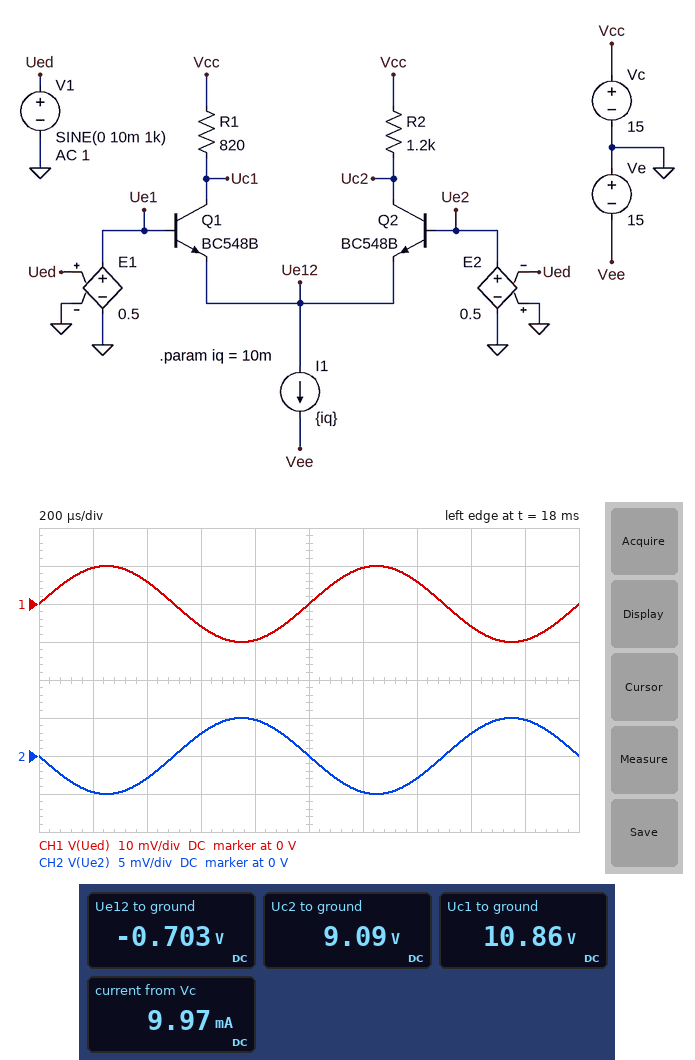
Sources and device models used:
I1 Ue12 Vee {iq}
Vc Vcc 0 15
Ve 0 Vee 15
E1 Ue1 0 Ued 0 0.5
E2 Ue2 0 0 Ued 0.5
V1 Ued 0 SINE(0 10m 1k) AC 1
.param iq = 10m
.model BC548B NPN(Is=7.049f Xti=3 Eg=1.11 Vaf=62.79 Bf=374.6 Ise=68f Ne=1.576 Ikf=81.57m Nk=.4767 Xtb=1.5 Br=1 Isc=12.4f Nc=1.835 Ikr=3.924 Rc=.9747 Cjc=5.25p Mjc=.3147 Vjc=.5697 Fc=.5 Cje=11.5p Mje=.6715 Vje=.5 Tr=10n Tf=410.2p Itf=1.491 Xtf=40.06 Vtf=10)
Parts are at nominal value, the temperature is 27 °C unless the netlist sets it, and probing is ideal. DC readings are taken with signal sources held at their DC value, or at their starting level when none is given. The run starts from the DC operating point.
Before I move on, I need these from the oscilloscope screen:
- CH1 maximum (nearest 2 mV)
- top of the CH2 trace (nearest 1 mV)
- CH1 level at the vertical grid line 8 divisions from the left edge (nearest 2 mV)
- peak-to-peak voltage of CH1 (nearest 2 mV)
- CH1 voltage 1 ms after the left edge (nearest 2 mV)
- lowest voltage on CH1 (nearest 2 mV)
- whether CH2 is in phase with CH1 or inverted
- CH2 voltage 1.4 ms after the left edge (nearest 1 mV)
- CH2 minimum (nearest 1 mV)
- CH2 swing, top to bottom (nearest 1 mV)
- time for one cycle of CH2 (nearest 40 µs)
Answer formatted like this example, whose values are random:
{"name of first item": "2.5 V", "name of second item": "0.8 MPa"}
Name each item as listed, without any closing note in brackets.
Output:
{"CH1 maximum": "10 mV", "top of the CH2 trace": "5 mV", "CH1 level at the vertical grid line 8 divisions from the left edge": "-6 mV", "peak-to-peak voltage of CH1": "20 mV", "CH1 voltage 1 ms after the left edge": "0 V", "lowest voltage on CH1": "-10 mV", "whether CH2 is in phase with CH1 or inverted": "inverted", "CH2 voltage 1.4 ms after the left edge": "-3 mV", "CH2 minimum": "-5 mV", "CH2 swing, top to bottom": "10 mV", "time for one cycle of CH2": "1.00 ms"}
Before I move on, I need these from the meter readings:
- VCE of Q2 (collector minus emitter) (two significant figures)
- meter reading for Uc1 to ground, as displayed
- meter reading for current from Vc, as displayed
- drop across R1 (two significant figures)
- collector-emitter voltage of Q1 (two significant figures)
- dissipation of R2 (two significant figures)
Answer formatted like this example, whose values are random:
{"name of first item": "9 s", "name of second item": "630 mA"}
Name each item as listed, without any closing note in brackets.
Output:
{"VCE of Q2 (collector minus emitter)": "9.8 V", "meter reading for Uc1 to ground, as displayed": "10.86 V", "meter reading for current from Vc, as displayed": "9.97 mA", "drop across R1": "4.1 V", "collector-emitter voltage of Q1": "12 V", "dissipation of R2": "29 mW"}
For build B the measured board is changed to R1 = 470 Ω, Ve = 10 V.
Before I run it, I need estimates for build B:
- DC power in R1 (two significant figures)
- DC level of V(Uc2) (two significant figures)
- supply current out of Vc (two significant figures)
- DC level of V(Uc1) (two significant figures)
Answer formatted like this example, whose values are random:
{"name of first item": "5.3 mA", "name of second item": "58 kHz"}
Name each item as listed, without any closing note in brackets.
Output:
{"DC power in R1": "12 mW", "DC level of V(Uc2)": "9.2 V", "supply current out of Vc": "10 mA", "DC level of V(Uc1)": "13 V"}
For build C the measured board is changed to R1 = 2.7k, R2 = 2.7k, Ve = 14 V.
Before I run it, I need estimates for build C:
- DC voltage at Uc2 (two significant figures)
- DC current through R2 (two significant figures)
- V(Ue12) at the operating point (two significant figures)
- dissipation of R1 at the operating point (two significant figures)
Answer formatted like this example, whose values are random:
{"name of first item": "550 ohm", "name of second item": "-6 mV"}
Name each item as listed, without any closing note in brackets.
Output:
{"DC voltage at Uc2": "1.5 V", "DC current through R2": "5.0 mA", "V(Ue12) at the operating point": "-710 mV", "dissipation of R1 at the operating point": "67 mW"}
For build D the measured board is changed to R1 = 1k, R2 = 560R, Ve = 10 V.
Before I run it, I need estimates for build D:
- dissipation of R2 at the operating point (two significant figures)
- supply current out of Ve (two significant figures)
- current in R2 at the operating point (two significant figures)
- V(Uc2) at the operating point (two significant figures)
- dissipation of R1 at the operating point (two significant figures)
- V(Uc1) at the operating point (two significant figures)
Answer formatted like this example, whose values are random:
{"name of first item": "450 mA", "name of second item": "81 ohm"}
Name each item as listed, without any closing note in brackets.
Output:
{"dissipation of R2 at the operating point": "14 mW", "supply current out of Ve": "10 mA", "current in R2 at the operating point": "5.1 mA", "V(Uc2) at the operating point": "12 V", "dissipation of R1 at the operating point": "24 mW", "V(Uc1) at the operating point": "10 V"}
